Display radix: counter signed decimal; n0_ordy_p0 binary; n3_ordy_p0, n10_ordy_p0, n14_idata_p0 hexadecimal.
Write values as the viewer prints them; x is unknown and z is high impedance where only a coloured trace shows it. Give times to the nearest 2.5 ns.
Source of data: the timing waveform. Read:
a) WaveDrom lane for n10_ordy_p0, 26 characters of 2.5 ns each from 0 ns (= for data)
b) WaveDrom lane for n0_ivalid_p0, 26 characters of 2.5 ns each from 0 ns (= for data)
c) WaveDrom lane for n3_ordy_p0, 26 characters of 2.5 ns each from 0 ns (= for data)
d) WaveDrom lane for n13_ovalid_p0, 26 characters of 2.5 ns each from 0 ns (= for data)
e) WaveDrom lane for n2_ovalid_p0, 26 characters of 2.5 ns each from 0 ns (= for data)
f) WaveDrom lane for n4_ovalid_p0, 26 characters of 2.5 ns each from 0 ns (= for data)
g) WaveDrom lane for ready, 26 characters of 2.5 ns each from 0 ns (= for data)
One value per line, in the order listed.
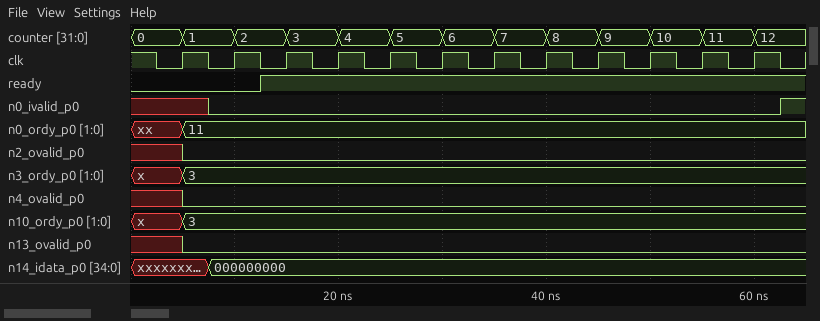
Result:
{name: 'n10_ordy_p0', wave: 'x.=.......................', data: '3'}
{name: 'n0_ivalid_p0', wave: 'x..0.....................1'}
{name: 'n3_ordy_p0', wave: 'x.=.......................', data: '3'}
{name: 'n13_ovalid_p0', wave: 'x.0.......................'}
{name: 'n2_ovalid_p0', wave: 'x.0.......................'}
{name: 'n4_ovalid_p0', wave: 'x.0.......................'}
{name: 'ready', wave: '0....1....................'}
